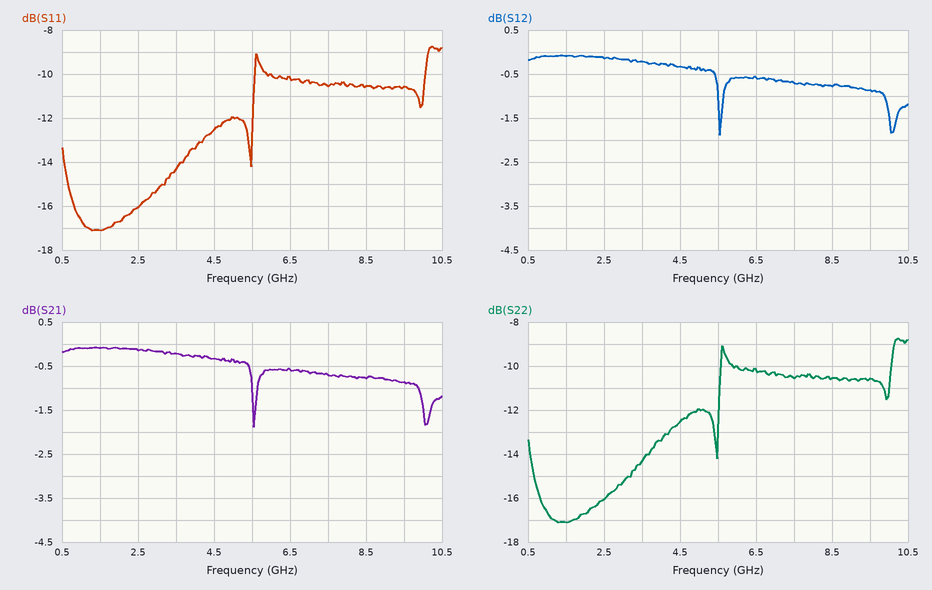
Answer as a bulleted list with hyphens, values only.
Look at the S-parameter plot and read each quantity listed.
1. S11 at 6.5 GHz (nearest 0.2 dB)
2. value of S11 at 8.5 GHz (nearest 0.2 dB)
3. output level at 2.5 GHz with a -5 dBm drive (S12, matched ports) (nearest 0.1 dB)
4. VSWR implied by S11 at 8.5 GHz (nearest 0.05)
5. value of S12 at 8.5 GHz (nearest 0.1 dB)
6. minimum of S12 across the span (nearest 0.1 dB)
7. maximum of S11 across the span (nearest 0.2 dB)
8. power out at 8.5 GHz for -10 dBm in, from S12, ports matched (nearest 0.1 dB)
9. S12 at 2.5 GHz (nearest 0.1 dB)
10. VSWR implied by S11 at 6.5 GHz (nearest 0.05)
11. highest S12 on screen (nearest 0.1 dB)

- -10.2 dB
- -10.6 dB
- -5.1 dBm
- 1.85
- -0.8 dB
- -1.9 dB
- -8.8 dB
- -10.8 dBm
- -0.1 dB
- 1.90
- -0.1 dB
